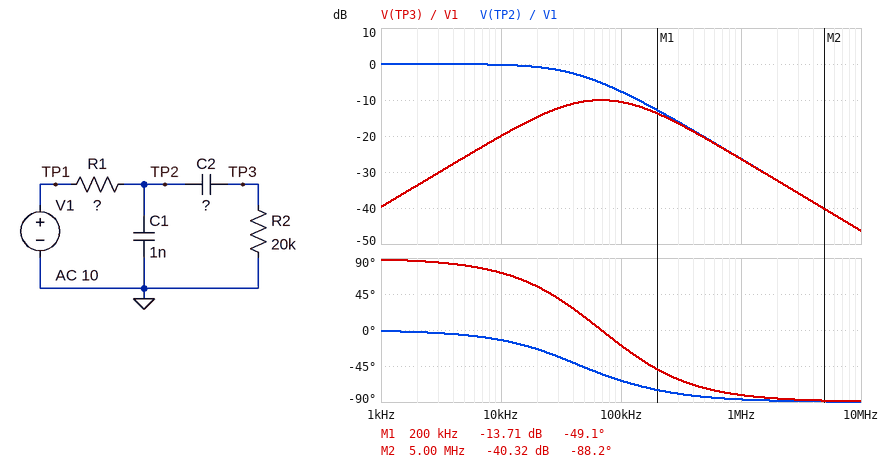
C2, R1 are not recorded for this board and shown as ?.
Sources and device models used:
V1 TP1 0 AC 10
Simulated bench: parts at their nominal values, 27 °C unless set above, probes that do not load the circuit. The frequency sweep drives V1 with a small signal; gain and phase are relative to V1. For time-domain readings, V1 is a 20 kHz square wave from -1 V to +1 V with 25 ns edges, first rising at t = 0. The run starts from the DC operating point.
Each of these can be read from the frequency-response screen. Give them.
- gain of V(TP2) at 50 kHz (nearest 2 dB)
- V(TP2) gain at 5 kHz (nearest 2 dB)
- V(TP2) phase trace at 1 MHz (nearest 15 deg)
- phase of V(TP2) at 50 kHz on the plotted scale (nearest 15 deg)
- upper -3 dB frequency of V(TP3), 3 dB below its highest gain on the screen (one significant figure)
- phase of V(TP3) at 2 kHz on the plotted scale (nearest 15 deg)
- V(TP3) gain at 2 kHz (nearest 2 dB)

-4 dB
0 dB
-90 deg
-45 deg
200 kHz
90 deg
-34 dB
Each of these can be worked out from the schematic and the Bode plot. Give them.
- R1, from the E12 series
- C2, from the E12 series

3.3 kΩ
82 pF
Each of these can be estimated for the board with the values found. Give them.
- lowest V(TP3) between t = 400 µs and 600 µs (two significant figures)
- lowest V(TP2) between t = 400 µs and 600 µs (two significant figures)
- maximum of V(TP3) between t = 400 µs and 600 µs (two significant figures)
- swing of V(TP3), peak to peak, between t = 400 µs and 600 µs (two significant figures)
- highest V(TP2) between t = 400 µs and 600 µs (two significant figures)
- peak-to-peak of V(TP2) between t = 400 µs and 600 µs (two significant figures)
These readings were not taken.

-480 mV
-1.0 V
480 mV
960 mV
1.0 V
2.0 V
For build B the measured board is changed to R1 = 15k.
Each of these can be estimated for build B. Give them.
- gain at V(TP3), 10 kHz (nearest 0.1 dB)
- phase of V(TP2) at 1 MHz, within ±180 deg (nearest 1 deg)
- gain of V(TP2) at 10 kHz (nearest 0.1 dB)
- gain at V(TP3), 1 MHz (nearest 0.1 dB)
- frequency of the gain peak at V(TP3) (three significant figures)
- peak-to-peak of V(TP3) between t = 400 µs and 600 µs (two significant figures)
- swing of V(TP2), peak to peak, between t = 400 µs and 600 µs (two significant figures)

-22.9 dB
-89 deg
-3.1 dB
-39.5 dB
32.1 kHz
250 mV
1.3 V
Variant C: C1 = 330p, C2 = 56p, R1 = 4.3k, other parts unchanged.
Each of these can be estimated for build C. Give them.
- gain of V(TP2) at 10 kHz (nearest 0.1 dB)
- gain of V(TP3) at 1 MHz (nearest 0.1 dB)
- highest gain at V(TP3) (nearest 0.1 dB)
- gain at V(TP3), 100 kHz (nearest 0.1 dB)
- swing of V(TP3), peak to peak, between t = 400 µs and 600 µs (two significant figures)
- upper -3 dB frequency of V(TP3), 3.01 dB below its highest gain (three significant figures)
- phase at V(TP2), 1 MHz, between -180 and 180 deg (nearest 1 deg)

-0.1 dB
-19.2 dB
-7.9 dB
-8.1 dB
1.2 V
327 kHz
-82 deg
